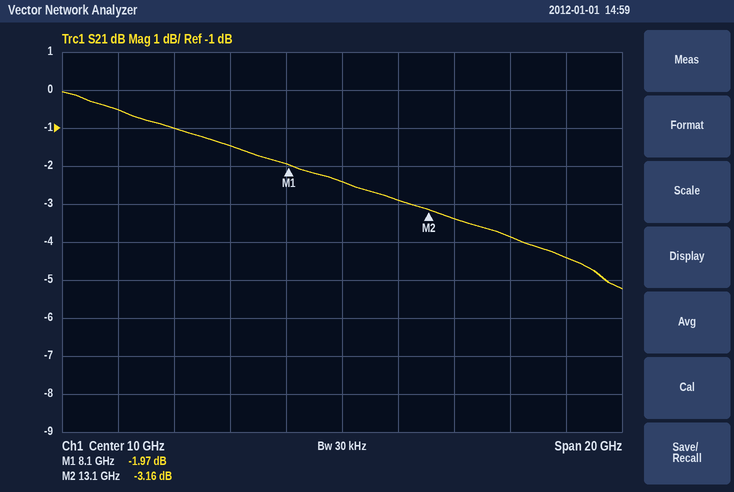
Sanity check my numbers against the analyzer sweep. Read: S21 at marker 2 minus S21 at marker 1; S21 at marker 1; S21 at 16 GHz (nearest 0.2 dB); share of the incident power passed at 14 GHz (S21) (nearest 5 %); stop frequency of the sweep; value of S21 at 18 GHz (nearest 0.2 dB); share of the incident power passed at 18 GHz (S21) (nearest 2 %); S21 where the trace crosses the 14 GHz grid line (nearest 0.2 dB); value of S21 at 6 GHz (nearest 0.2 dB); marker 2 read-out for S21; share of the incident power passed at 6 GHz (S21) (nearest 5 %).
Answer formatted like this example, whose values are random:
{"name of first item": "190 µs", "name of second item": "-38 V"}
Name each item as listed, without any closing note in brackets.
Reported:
{"S21 at marker 2 minus S21 at marker 1": "-1.19 dB", "S21 at marker 1": "-1.97 dB", "S21 at 16 GHz": "-3.8 dB", "share of the incident power passed at 14 GHz (S21)": "45 %", "stop frequency of the sweep": "20 GHz", "value of S21 at 18 GHz": "-4.4 dB", "share of the incident power passed at 18 GHz (S21)": "36 %", "S21 where the trace crosses the 14 GHz grid line": "-3.4 dB", "value of S21 at 6 GHz": "-1.4 dB", "marker 2 read-out for S21": "-3.16 dB", "share of the incident power passed at 6 GHz (S21)": "70 %"}
